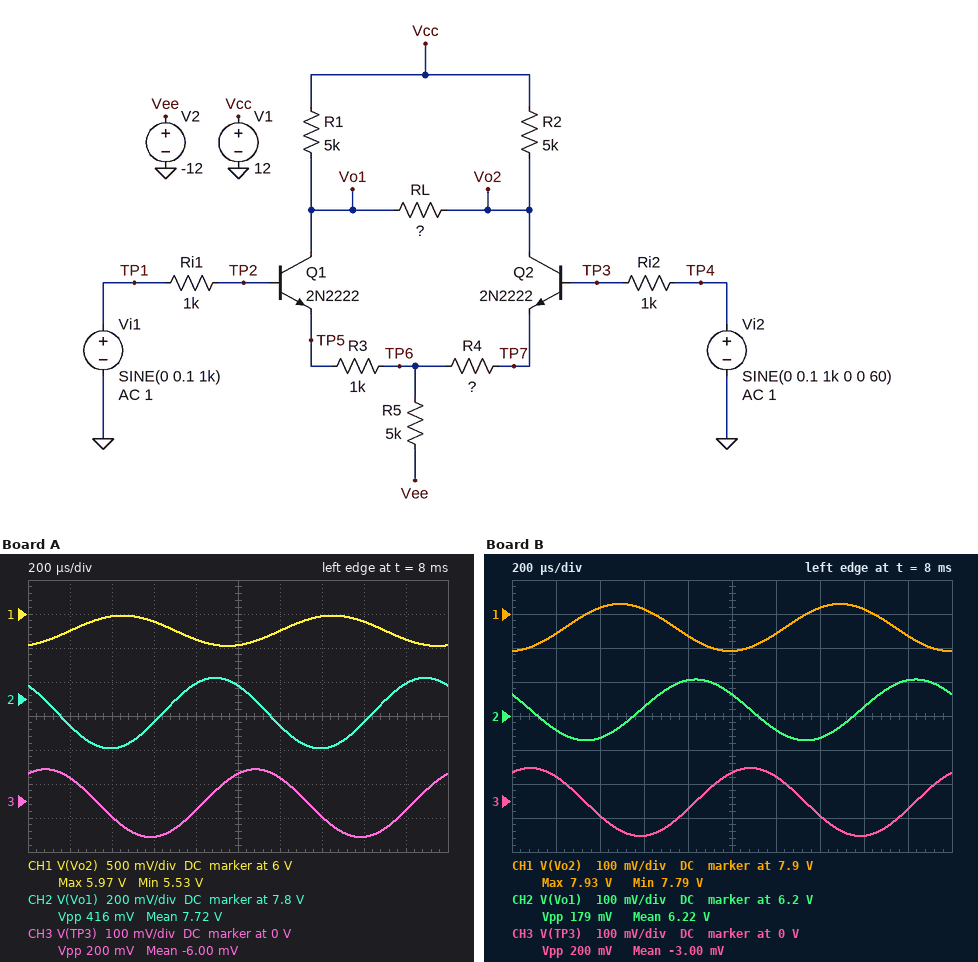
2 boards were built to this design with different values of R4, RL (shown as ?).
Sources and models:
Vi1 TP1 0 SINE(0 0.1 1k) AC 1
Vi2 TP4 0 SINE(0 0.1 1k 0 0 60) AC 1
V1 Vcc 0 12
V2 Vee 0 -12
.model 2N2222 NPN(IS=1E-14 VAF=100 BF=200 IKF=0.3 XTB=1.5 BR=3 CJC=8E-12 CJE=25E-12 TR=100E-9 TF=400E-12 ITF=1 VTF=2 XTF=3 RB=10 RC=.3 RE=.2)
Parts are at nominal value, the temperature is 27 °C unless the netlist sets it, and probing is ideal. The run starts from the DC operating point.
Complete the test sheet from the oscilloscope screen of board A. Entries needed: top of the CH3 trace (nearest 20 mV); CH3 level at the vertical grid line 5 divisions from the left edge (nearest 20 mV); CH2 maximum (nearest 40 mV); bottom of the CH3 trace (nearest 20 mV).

100 mV
80 mV
7.92 V
-100 mV
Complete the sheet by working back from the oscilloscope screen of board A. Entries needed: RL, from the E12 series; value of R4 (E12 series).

22 kΩ
560 Ω
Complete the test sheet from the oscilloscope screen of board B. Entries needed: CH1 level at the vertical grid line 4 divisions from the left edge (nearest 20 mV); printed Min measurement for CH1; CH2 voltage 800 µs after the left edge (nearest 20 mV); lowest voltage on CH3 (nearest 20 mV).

7.84 V
7.79 V
6.30 V
-100 mV
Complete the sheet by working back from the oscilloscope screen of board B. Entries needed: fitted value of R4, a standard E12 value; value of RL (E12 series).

2.2 kΩ
8.2 kΩ
